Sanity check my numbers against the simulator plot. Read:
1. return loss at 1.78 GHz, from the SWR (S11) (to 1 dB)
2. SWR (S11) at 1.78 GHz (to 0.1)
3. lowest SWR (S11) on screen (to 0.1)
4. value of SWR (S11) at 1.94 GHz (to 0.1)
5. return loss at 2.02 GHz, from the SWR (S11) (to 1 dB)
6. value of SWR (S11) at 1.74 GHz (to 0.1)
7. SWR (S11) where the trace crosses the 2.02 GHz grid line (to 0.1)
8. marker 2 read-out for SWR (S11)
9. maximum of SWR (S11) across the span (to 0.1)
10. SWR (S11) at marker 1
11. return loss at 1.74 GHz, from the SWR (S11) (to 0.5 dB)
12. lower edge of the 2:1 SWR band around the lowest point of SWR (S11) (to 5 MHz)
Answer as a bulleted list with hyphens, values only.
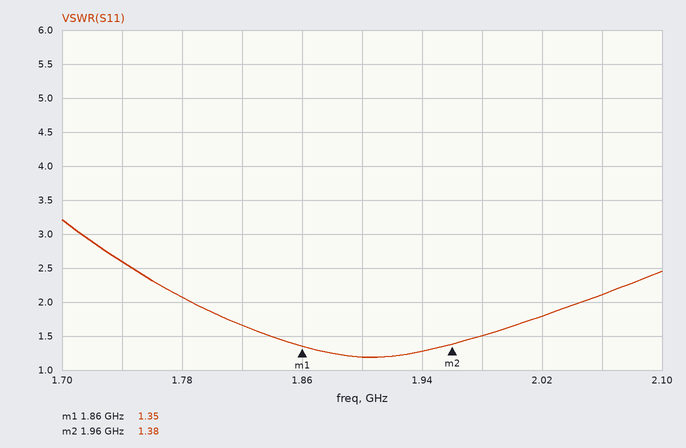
- 9 dB
- 2.1
- 1.2
- 1.3
- 11 dB
- 2.6
- 1.8
- 1.38
- 3.2
- 1.35
- 7.0 dB
- 1.785 GHz
